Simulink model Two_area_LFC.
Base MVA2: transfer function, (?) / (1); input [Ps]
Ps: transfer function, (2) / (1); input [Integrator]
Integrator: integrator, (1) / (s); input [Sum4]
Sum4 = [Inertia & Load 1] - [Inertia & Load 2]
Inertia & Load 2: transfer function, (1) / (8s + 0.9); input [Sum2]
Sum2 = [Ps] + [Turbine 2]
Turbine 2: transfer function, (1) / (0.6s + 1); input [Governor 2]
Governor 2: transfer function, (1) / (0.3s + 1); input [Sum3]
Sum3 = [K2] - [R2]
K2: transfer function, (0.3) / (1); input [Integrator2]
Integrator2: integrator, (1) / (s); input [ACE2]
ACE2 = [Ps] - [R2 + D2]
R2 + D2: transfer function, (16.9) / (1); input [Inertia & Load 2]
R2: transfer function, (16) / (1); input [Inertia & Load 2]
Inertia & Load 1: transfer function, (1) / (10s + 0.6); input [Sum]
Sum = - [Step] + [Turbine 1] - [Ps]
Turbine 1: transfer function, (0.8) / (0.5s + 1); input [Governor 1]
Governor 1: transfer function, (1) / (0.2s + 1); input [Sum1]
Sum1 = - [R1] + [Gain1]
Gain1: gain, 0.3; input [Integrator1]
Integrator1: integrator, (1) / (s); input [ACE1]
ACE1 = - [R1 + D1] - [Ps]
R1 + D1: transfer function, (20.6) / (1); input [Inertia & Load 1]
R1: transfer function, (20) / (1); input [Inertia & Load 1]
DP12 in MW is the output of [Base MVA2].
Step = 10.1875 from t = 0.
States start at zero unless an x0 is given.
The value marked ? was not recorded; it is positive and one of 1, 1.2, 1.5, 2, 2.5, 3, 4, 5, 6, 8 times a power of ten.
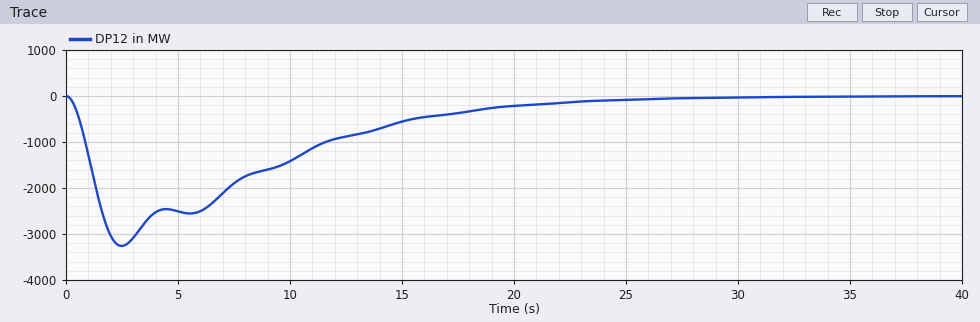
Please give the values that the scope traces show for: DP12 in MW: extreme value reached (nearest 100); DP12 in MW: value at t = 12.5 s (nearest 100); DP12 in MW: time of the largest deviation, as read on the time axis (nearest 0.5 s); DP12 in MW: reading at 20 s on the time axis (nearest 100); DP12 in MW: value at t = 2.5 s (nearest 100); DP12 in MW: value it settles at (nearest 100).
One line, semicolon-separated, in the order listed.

-3300; -900; 2.5 s; -200; -3300; 0
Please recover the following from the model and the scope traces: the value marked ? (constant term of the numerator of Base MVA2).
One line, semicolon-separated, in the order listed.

1500
